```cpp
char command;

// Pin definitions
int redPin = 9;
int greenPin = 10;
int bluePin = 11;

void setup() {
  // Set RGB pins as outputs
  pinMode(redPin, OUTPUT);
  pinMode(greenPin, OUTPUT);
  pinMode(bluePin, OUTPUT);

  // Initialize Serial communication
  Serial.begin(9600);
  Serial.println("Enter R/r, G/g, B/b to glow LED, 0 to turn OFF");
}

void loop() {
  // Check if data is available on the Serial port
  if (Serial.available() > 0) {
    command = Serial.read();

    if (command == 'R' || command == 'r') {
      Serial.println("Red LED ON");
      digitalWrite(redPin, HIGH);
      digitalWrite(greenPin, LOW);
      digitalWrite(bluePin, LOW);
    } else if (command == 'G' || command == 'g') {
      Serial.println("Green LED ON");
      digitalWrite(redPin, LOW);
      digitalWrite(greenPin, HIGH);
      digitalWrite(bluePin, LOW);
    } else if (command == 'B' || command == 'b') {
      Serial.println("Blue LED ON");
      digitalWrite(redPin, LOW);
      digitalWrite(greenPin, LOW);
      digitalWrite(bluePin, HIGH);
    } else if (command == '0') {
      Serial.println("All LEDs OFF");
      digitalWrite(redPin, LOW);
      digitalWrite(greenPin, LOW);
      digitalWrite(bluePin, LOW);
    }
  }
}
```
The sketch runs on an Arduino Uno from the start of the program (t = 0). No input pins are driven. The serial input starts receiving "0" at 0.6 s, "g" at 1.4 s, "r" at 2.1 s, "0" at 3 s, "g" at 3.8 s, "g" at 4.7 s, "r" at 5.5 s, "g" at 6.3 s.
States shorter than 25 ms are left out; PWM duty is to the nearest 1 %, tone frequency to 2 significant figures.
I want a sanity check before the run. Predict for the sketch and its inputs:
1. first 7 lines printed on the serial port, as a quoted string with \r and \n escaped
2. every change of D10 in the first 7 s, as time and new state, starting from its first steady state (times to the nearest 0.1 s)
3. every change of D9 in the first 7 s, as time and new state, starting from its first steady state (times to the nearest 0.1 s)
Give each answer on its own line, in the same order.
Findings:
"Enter R/r, G/g, B/b to glow LED, 0 to turn OFF\r\nAll LEDs OFF\r\nGreen LED ON\r\nRed LED ON\r\nAll LEDs OFF\r\nGreen LED ON\r\nGreen LED ON\r\n"
0 s low; 1.4 s high; 2.1 s low; 3.8 s high; 5.5 s low; 6.3 s high
0 s low; 2.1 s high; 3 s low; 5.5 s high; 6.3 s low
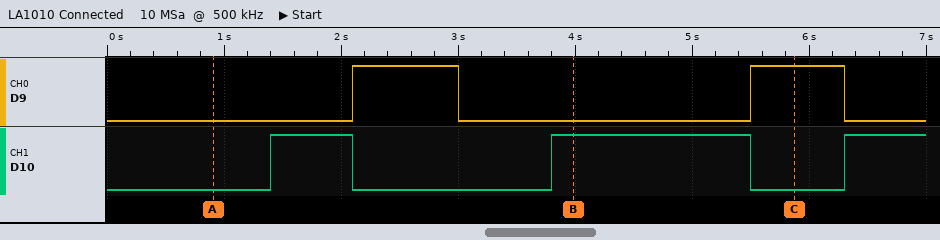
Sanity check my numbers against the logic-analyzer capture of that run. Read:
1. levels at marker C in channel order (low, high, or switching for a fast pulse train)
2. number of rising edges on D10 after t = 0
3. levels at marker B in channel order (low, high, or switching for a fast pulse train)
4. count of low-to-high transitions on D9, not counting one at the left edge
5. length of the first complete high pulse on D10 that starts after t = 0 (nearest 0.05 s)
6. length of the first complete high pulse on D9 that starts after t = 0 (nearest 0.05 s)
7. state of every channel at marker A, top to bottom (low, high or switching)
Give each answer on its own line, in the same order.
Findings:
D9 high, D10 low
3
D9 low, D10 high
2
0.70 s
0.90 s
D9 low, D10 low
